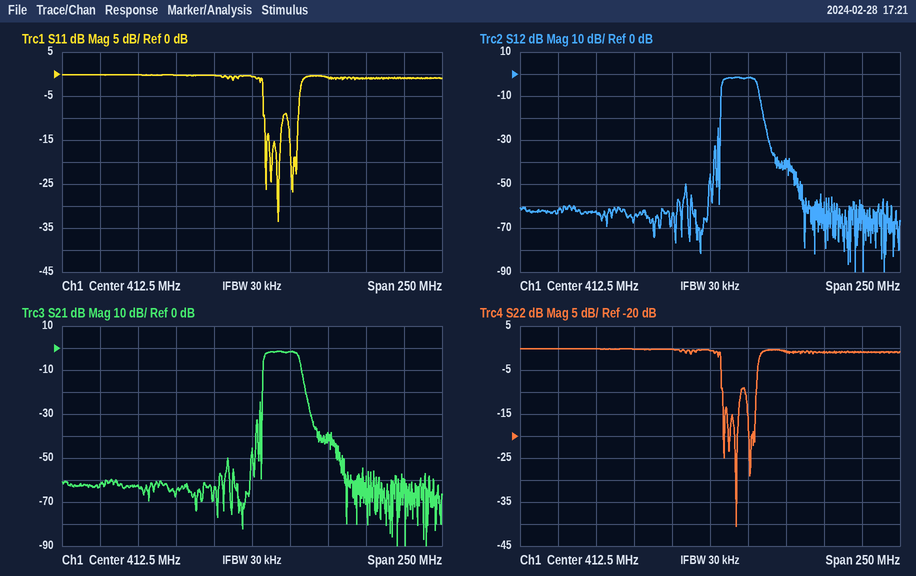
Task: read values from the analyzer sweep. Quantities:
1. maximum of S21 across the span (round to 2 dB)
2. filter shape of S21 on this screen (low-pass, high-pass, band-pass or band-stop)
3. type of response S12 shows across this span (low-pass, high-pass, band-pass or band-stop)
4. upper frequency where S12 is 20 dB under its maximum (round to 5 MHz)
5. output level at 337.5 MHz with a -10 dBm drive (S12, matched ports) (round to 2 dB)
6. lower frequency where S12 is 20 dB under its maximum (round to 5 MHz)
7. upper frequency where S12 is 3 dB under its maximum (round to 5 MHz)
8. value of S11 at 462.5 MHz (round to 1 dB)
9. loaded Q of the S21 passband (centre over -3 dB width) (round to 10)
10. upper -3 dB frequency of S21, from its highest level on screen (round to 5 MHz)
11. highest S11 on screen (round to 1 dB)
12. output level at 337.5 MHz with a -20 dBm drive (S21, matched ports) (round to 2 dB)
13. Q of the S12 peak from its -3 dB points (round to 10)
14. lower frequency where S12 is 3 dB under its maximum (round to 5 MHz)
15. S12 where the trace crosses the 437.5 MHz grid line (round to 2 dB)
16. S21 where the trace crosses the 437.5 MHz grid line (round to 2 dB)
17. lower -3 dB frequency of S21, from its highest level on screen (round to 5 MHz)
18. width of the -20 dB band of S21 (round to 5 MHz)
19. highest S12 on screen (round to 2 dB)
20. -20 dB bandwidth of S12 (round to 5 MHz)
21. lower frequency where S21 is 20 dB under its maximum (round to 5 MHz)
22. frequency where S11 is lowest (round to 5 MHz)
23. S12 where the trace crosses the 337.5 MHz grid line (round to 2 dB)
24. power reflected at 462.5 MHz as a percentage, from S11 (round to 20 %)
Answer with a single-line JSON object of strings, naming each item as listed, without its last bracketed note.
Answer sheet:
{"maximum of S21 across the span": "-2 dB", "filter shape of S21 on this screen": "band-pass", "type of response S12 shows across this span": "band-pass", "upper frequency where S12 is 20 dB under its maximum": "450 MHz", "output level at 337.5 MHz with a -10 dBm drive (S12, matched ports)": "-72 dBm", "lower frequency where S12 is 20 dB under its maximum": "420 MHz", "upper frequency where S12 is 3 dB under its maximum": "445 MHz", "value of S11 at 462.5 MHz": "-1 dB", "loaded Q of the S21 passband (centre over -3 dB width)": "20", "upper -3 dB frequency of S21, from its highest level on screen": "445 MHz", "highest S11 on screen": "0 dB", "output level at 337.5 MHz with a -20 dBm drive (S21, matched ports)": "-82 dBm", "Q of the S12 peak from its -3 dB points": "20", "lower frequency where S12 is 3 dB under its maximum": "420 MHz", "S12 where the trace crosses the 437.5 MHz grid line": "-2 dB", "S21 where the trace crosses the 437.5 MHz grid line": "-2 dB", "lower -3 dB frequency of S21, from its highest level on screen": "420 MHz", "width of the -20 dB band of S21": "30 MHz", "highest S12 on screen": "-2 dB", "-20 dB bandwidth of S12": "30 MHz", "lower frequency where S21 is 20 dB under its maximum": "420 MHz", "frequency where S11 is lowest": "430 MHz", "S12 where the trace crosses the 337.5 MHz grid line": "-62 dB", "power reflected at 462.5 MHz as a percentage, from S11": "80 %"}
